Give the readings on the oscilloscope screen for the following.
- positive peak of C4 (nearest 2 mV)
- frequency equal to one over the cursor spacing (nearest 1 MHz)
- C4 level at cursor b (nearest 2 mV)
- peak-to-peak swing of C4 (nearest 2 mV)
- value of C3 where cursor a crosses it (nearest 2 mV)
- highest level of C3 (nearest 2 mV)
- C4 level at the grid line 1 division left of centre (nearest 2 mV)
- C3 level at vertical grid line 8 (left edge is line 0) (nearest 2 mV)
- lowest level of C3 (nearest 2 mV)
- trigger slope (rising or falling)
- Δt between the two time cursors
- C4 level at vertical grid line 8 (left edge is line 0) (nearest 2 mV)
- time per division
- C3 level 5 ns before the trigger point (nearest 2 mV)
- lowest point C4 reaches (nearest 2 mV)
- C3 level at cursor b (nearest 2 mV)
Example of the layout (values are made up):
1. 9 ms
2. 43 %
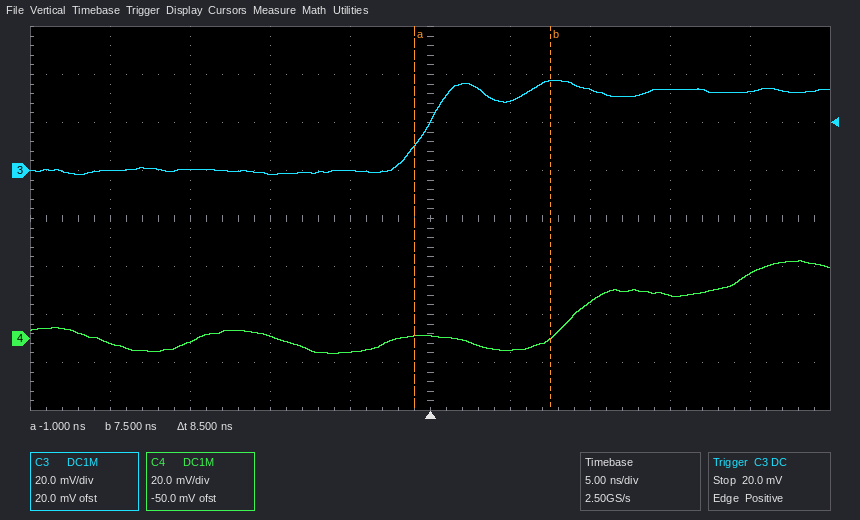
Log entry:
1. 32 mV
2. 118 MHz
3. 0 mV
4. 38 mV
5. 10 mV
6. 38 mV
7. -6 mV
8. 34 mV
9. -2 mV
10. rising
11. 8.5 ns
12. 18 mV
13. 5 ns
14. 0 mV
15. -6 mV
16. 38 mV
